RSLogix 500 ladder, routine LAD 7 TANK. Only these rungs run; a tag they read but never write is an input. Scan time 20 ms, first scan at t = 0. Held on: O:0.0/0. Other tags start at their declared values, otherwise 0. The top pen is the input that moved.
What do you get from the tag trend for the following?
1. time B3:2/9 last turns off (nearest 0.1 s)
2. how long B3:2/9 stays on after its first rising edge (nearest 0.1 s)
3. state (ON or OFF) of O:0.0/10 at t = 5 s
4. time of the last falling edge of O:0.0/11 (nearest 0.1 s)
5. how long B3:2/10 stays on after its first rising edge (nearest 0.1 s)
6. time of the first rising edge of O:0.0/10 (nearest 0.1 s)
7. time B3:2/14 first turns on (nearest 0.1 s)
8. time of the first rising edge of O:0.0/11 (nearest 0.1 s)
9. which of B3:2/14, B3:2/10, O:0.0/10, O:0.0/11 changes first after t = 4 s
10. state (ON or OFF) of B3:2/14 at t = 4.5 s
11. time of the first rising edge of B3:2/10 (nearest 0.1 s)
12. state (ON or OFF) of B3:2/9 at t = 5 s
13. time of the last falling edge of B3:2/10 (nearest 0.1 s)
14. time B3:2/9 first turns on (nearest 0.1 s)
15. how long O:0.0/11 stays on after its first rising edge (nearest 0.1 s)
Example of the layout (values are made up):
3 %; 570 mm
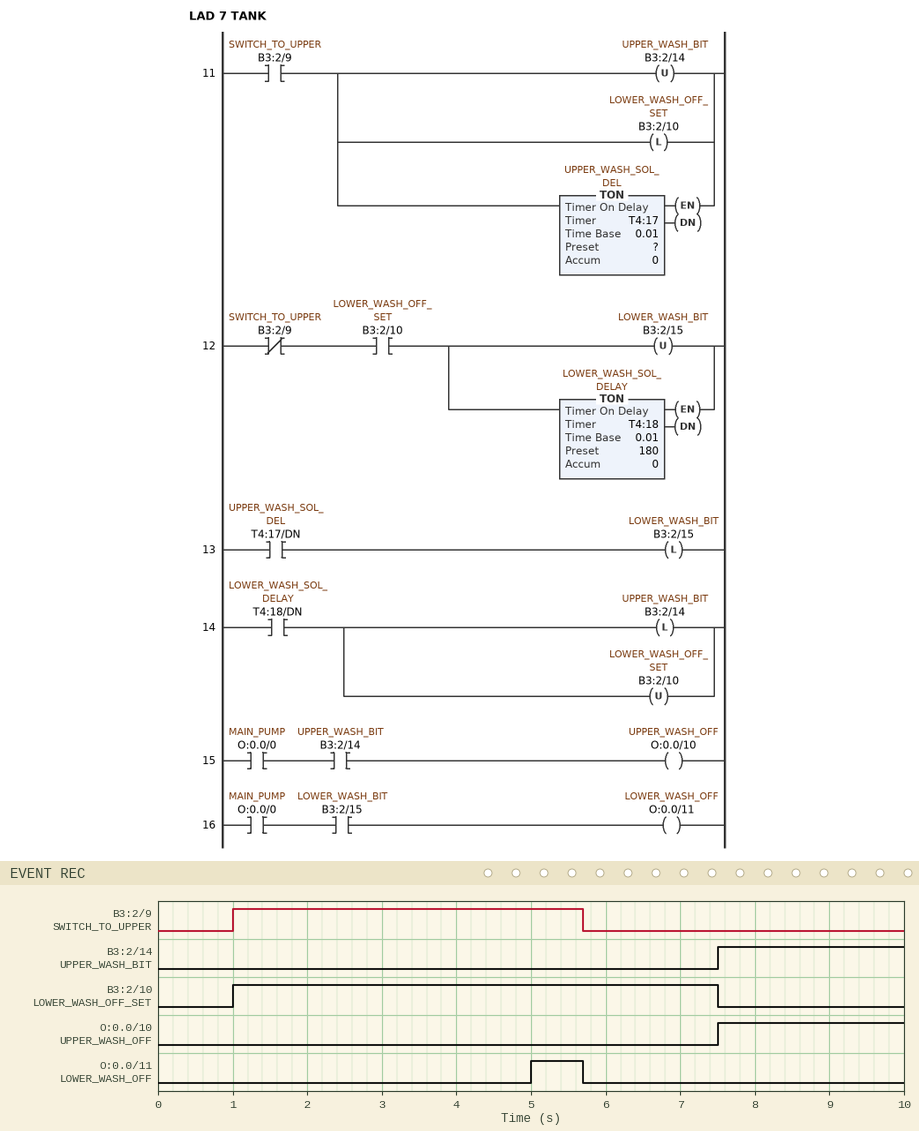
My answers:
5.7 s; 4.7 s; OFF; 5.7 s; 6.5 s; 7.5 s; 7.5 s; 5.0 s; O:0.0/11; OFF; 1.0 s; ON; 7.5 s; 1.0 s; 0.7 s
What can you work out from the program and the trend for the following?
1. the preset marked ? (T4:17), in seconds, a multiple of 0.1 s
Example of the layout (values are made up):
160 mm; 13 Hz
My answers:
4.0 s
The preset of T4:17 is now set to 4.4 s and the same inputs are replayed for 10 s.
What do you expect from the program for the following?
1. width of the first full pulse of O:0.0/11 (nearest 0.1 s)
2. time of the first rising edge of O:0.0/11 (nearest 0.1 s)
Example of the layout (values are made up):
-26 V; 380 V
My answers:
0.3 s; 5.4 s
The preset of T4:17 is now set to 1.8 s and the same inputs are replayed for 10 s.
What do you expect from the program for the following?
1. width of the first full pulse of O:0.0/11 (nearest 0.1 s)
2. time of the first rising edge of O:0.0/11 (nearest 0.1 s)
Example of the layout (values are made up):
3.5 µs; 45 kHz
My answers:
2.9 s; 2.8 s
